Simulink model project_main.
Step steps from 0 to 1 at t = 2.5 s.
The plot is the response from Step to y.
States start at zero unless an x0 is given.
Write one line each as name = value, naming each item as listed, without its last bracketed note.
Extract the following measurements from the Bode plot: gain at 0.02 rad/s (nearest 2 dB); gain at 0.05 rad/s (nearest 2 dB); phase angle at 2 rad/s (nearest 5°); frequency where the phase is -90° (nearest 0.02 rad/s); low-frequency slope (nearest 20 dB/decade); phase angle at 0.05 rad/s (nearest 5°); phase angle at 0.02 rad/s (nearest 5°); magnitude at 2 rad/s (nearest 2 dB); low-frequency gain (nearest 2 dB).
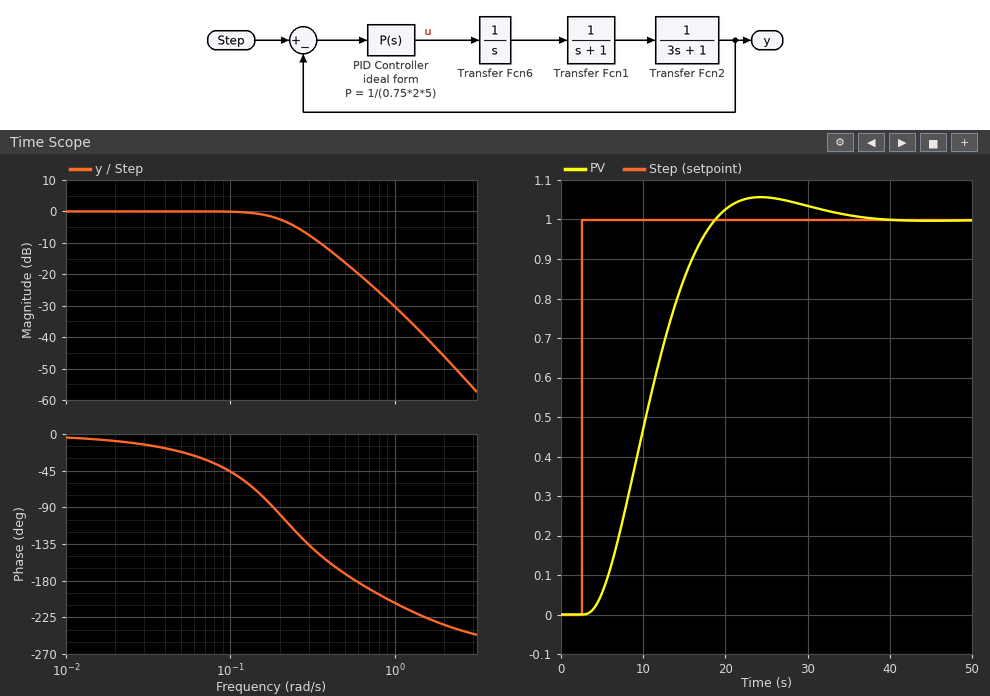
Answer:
gain at 0.02 rad/s = 0 dB
gain at 0.05 rad/s = 0 dB
phase angle at 2 rad/s = -235°
frequency where the phase is -90° = 0.18 rad/s
low-frequency slope = 0 dB/decade
phase angle at 0.05 rad/s = -20°
phase angle at 0.02 rad/s = -10°
magnitude at 2 rad/s = -46 dB
low-frequency gain = 0 dB
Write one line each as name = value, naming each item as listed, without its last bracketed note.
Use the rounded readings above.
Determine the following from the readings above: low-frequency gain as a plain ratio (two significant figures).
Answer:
low-frequency gain as a plain ratio = 1.0
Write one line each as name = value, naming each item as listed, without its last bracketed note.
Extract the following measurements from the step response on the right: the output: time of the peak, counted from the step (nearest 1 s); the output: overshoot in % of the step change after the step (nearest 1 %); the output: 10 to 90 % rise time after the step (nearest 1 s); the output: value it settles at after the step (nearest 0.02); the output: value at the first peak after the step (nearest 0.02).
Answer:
the output: time of the peak, counted from the step = 22 s
the output: overshoot in % of the step change after the step = 6 %
the output: 10 to 90 % rise time after the step = 10 s
the output: value it settles at after the step = 1.00
the output: value at the first peak after the step = 1.06
